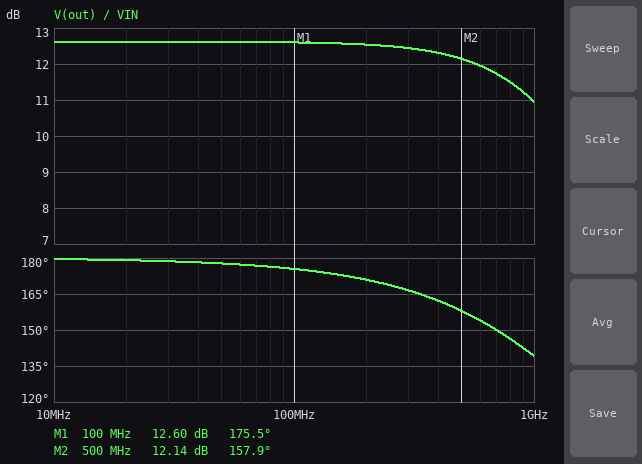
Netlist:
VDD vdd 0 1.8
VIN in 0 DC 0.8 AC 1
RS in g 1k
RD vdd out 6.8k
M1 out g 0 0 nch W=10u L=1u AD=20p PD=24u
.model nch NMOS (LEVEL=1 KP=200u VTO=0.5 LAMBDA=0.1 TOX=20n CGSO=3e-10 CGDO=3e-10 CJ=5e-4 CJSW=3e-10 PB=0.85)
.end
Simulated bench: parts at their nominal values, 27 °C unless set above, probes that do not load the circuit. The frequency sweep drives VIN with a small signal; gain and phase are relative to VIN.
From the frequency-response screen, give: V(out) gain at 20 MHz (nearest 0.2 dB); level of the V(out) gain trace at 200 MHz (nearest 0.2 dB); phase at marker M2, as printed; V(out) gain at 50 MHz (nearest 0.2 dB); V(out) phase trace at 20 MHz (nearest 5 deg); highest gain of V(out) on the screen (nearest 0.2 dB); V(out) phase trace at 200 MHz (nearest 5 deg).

12.6 dB
12.6 dB
157.9 deg
12.6 dB
180 deg
12.6 dB
170 deg
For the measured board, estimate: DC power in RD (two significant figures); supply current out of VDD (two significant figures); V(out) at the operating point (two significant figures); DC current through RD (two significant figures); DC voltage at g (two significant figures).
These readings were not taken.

68 µW
100 µA
1.1 V
100 µA
800 mV
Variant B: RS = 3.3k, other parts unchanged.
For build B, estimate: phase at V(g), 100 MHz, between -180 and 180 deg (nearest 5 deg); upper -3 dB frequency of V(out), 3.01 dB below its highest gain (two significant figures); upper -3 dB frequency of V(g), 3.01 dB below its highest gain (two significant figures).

-5 deg
960 MHz
1.5 GHz
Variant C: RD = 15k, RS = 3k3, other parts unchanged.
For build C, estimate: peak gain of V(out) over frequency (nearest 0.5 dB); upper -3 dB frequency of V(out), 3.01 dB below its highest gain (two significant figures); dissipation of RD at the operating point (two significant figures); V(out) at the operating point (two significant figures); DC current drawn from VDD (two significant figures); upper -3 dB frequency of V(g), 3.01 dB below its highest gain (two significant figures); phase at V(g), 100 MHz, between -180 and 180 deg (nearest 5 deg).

18.5 dB
480 MHz
130 µW
400 mV
94 µA
1.3 GHz
-5 deg
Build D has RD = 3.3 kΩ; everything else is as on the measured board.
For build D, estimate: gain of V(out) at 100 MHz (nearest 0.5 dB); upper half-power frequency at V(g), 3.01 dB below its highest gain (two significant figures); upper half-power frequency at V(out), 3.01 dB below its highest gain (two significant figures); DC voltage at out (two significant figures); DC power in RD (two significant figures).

7.0 dB
7.3 GHz
2.8 GHz
1.5 V
35 µW
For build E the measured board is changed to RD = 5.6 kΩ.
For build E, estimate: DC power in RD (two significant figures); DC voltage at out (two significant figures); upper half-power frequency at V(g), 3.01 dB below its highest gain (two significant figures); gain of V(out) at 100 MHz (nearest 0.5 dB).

57 µW
1.2 V
7.5 GHz
11.0 dB
